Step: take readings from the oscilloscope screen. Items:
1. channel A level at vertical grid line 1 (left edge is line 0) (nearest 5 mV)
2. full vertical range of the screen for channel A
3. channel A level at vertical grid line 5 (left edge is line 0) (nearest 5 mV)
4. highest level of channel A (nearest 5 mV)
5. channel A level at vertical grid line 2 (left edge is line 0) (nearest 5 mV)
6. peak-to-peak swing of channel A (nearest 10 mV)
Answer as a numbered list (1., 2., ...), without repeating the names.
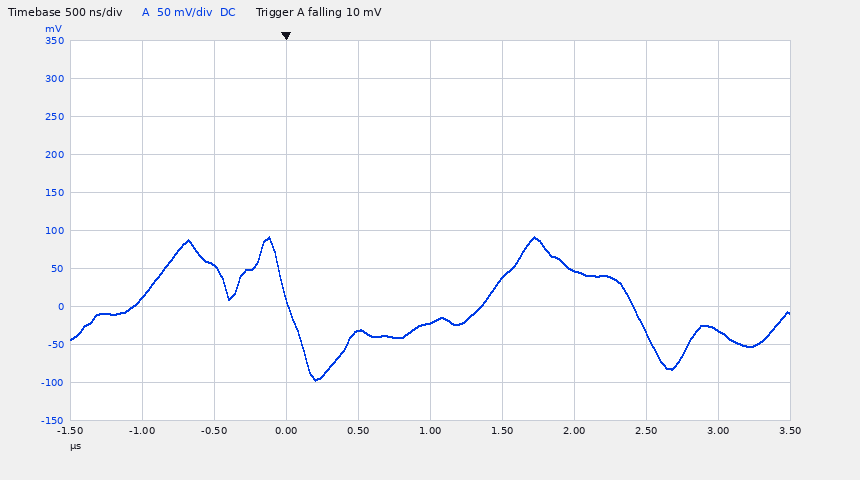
1. 10 mV
2. 500 mV
3. -20 mV
4. 90 mV
5. 55 mV
6. 190 mV
